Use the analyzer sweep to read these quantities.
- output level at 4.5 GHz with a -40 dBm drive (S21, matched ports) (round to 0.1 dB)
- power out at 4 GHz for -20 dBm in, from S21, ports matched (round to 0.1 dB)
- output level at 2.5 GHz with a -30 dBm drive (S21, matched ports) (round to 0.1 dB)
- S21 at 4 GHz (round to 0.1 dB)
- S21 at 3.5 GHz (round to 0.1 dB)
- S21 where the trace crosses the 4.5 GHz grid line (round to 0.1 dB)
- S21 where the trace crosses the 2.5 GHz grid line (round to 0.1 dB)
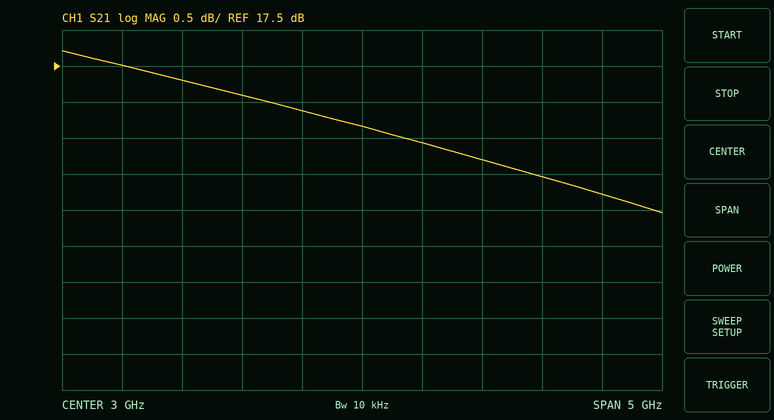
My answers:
-24.0 dBm
-3.8 dBm
-13.1 dBm
16.2 dB
16.4 dB
16.0 dB
16.9 dB
